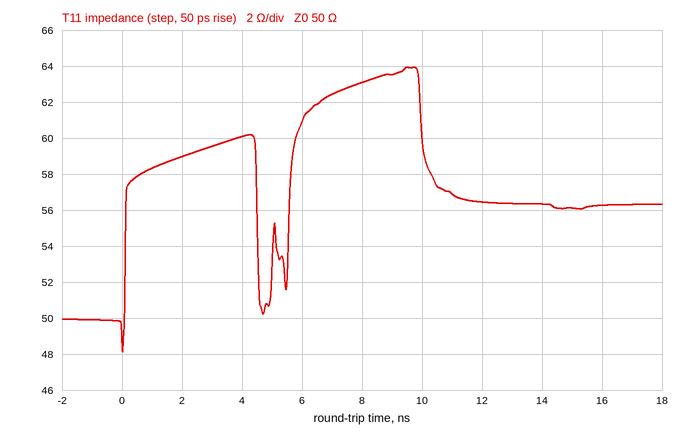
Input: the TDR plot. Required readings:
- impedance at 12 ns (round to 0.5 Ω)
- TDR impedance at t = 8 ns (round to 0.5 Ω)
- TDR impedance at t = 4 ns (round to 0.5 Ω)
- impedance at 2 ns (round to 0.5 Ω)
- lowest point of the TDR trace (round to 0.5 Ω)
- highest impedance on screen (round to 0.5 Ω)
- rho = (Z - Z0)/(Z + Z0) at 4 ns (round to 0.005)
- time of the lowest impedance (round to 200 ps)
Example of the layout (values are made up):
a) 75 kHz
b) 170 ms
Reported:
a) 56.5 Ω
b) 63.0 Ω
c) 60.0 Ω
d) 59.0 Ω
e) 48.0 Ω
f) 64.0 Ω
g) +0.090
h) 0.0 ns
